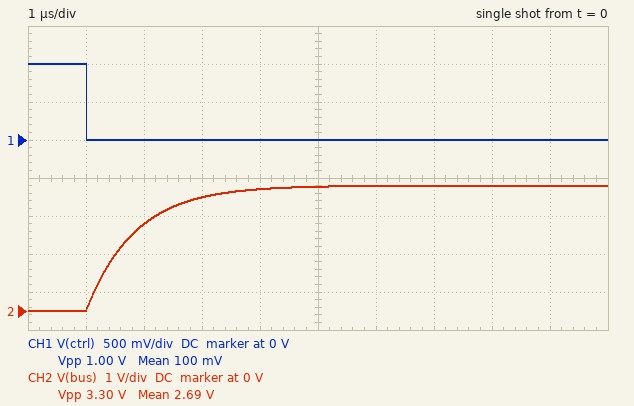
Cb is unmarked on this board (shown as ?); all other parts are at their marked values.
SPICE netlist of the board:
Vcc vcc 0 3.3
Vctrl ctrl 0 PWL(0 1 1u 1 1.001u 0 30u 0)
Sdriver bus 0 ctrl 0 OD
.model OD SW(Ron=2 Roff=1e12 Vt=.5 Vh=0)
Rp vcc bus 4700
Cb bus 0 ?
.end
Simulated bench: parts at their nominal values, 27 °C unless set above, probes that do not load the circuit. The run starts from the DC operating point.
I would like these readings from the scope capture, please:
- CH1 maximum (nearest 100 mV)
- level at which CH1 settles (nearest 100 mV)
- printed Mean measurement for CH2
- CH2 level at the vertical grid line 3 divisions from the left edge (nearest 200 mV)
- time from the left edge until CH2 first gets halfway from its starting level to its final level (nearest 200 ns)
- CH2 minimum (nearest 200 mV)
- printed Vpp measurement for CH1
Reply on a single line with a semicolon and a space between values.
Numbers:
1.0 V; 0 V; 2.69 V; 3.0 V; 1.6 µs; 0 V; 1.00 V
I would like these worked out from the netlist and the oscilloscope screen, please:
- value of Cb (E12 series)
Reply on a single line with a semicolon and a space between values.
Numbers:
180 pF
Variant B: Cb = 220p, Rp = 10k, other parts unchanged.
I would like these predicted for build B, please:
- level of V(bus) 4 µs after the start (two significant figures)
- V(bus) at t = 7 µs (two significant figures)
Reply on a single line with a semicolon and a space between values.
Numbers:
2.5 V; 3.1 V
